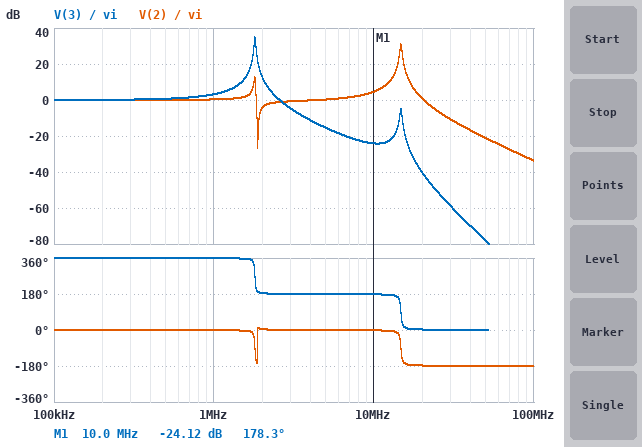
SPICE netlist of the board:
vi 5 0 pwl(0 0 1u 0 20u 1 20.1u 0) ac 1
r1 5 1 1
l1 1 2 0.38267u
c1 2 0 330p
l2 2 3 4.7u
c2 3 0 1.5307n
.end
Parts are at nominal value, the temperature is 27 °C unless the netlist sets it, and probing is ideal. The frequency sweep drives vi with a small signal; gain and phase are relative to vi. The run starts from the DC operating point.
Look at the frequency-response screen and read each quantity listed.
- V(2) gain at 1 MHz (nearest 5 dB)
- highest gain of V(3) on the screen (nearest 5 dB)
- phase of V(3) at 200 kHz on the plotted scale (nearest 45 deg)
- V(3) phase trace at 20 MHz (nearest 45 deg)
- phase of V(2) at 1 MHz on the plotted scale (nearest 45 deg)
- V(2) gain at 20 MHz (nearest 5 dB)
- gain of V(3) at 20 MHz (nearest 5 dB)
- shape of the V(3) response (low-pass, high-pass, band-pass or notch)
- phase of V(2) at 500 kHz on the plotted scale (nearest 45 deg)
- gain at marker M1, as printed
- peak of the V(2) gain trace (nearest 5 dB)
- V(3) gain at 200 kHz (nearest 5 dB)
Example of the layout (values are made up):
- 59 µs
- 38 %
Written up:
- 0 dB
- 35 dB
- 360 deg
- 0 deg
- 0 deg
- 0 dB
- -40 dB
- low-pass
- 0 deg
- -24.12 dB
- 30 dB
- 0 dB
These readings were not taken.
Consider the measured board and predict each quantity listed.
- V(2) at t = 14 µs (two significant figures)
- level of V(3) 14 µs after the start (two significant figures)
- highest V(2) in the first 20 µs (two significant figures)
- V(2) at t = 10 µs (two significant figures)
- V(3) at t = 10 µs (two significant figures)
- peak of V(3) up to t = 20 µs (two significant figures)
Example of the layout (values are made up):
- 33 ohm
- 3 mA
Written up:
- 680 mV
- 680 mV
- 1.0 V
- 470 mV
- 470 mV
- 1.0 V
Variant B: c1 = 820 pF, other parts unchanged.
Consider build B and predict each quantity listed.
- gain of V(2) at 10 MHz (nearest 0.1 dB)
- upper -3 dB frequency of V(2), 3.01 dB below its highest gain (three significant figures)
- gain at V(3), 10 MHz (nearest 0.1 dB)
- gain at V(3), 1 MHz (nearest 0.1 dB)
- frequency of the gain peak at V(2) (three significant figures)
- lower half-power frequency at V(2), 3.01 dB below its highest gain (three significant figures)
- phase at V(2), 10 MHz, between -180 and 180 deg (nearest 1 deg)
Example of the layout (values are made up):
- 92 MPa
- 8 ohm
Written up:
- 15.8 dB
- 9.54 MHz
- -12.9 dB
- 3.3 dB
- 9.35 MHz
- 9.16 MHz
- -163 deg
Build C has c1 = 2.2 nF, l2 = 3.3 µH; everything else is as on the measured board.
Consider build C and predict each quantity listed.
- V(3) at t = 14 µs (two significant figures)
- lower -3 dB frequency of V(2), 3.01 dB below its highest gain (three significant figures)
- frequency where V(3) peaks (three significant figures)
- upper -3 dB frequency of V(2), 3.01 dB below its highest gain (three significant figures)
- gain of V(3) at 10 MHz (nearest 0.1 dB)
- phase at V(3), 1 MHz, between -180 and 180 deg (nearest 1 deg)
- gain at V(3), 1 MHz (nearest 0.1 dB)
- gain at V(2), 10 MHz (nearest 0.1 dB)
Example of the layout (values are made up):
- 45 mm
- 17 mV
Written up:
- 680 mV
- 5.66 MHz
- 2.10 MHz
- 6.02 MHz
- -32.4 dB
- -2 deg
- 2.5 dB
- -6.9 dB
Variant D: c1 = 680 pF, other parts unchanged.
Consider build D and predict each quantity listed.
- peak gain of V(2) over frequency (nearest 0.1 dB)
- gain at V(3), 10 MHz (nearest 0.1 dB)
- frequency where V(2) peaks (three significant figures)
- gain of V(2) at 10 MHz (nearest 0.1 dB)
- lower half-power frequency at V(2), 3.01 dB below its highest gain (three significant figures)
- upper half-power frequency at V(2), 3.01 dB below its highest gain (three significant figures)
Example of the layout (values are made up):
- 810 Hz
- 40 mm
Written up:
- 27.9 dB
- -5.6 dB
- 10.3 MHz
- 23.2 dB
- 10.1 MHz
- 10.5 MHz
